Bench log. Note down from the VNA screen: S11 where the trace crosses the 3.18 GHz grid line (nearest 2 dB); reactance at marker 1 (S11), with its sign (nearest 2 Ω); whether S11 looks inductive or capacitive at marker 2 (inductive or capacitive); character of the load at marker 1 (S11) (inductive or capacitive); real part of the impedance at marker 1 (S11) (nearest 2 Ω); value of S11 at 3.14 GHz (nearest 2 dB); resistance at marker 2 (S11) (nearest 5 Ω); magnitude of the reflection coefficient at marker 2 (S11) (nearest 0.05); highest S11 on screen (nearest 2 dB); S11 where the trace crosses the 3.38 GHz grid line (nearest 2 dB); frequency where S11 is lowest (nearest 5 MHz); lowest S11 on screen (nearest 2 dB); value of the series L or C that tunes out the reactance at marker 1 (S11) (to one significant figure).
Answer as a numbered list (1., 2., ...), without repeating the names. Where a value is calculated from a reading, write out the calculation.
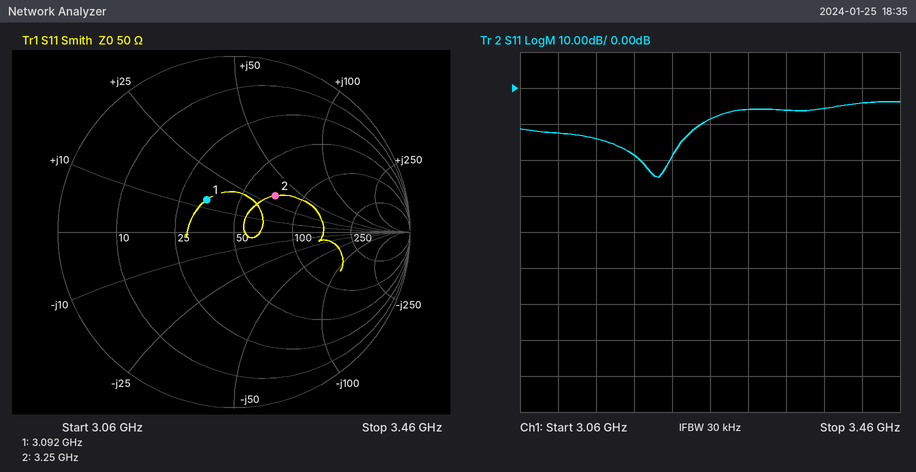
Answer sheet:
1. -18 dB
2. +14 Ω
3. inductive
4. inductive
5. 34 Ω
6. -14 dB
7. 70 Ω
8. 0.30
9. -4 dB
10. -6 dB
11. 3.205 GHz
12. -24 dB
13. C = 1/(2π × 3.092 GHz × 14 Ω) ≈ 4 pF
